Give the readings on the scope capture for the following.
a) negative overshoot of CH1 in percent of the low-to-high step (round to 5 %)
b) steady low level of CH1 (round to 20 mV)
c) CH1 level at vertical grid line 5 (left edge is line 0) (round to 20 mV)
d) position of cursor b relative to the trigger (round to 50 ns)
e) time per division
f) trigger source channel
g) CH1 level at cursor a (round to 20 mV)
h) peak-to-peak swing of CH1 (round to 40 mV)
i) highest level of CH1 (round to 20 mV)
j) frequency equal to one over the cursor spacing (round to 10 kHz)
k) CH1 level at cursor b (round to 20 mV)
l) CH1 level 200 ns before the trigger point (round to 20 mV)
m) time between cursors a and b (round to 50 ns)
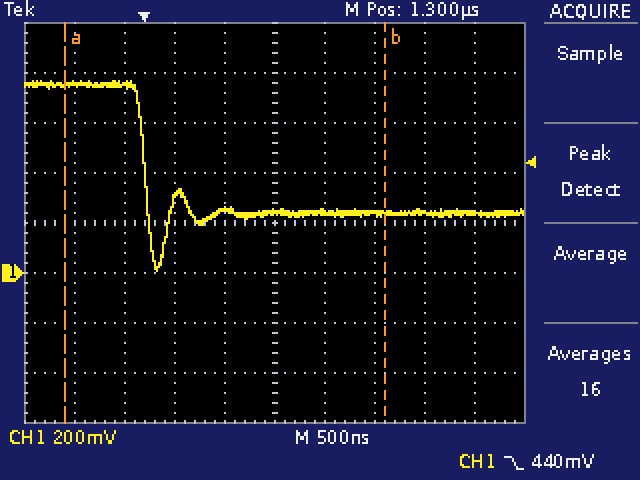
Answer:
45 %
240 mV
240 mV
+2.40 µs
500 ns
CH1
760 mV
760 mV
760 mV
310 kHz
240 mV
760 mV
3.20 µs
